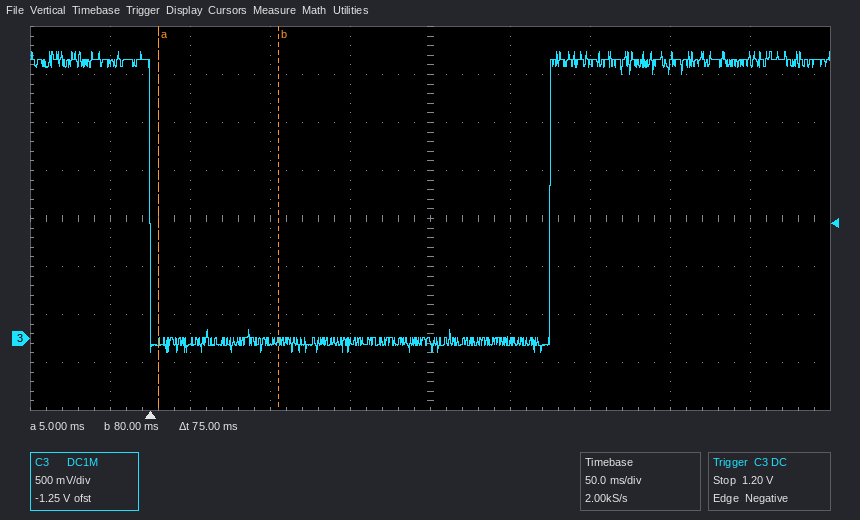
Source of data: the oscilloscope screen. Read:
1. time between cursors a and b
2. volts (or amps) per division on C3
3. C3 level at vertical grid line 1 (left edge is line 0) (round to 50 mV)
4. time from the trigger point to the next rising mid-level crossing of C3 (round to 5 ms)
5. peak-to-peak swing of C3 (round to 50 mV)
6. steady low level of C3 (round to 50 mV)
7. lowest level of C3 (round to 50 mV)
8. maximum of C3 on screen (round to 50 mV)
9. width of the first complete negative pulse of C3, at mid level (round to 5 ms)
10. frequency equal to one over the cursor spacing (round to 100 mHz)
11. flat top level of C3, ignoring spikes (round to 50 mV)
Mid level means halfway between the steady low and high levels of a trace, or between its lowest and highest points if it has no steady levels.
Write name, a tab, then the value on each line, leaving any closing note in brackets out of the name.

time between cursors a and b	75 ms
volts (or amps) per division on C3	500 mV
C3 level at vertical grid line 1 (left edge is line 0)	2.85 V
time from the trigger point to the next rising mid-level crossing of C3	250 ms
peak-to-peak swing of C3	3.15 V
steady low level of C3	-50 mV
lowest level of C3	-150 mV
maximum of C3 on screen	3.00 V
width of the first complete negative pulse of C3, at mid level	250 ms
frequency equal to one over the cursor spacing	13.3 Hz
flat top level of C3, ignoring spikes	2.90 V
